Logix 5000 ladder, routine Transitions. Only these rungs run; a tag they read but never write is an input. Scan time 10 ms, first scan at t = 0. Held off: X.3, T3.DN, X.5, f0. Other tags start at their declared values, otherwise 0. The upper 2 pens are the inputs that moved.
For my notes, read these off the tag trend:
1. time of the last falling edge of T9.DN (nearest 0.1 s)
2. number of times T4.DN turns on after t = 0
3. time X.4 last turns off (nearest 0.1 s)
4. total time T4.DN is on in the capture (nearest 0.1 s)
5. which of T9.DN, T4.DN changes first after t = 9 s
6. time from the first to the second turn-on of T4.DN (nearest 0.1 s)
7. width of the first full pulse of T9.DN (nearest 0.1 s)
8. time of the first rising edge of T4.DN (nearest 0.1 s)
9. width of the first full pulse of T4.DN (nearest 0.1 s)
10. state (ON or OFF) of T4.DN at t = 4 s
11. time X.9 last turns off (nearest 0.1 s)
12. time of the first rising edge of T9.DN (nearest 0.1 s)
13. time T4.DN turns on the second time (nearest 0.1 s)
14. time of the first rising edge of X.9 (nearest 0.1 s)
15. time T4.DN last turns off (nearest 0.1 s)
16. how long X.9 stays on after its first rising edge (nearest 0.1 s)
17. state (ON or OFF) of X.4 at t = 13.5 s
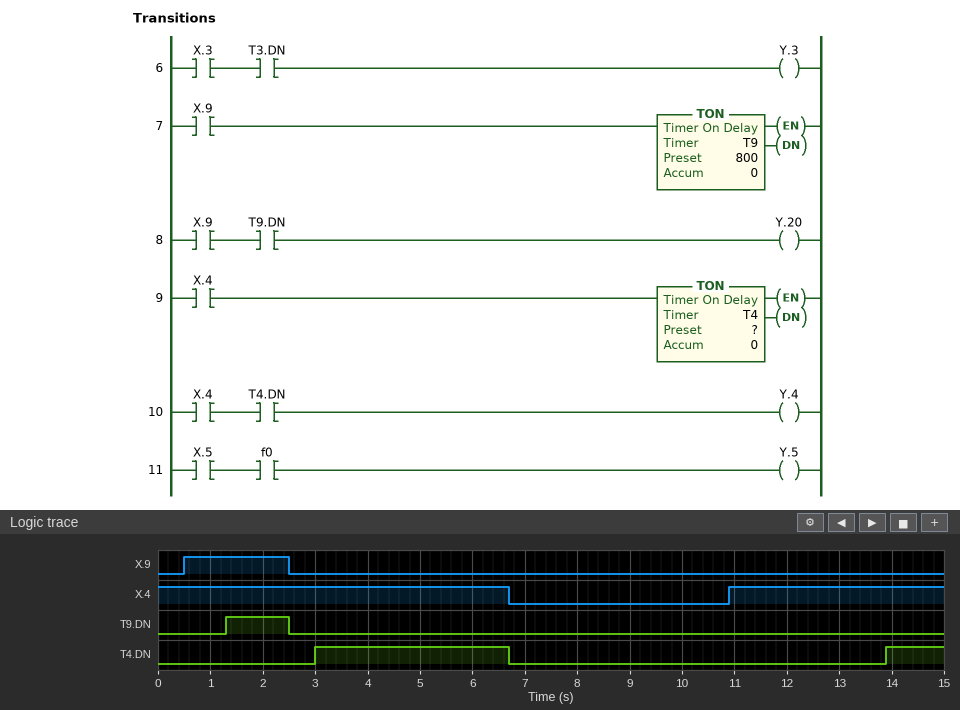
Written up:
2.5 s
2
6.7 s
4.8 s
T4.DN
10.9 s
1.2 s
3.0 s
3.7 s
ON
2.5 s
1.3 s
13.9 s
0.5 s
6.7 s
2.0 s
ON
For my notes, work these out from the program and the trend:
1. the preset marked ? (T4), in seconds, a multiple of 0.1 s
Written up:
3.0 s
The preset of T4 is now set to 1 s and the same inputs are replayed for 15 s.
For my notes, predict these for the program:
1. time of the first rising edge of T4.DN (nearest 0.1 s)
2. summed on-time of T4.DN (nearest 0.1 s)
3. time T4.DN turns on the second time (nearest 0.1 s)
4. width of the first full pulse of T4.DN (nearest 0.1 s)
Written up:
1.0 s
8.8 s
11.9 s
5.7 s
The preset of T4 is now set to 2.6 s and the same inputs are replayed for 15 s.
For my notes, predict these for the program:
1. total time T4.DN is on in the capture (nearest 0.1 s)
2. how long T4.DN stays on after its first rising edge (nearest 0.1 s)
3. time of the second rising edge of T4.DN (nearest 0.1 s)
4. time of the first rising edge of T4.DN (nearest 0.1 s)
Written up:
5.6 s
4.1 s
13.5 s
2.6 s
